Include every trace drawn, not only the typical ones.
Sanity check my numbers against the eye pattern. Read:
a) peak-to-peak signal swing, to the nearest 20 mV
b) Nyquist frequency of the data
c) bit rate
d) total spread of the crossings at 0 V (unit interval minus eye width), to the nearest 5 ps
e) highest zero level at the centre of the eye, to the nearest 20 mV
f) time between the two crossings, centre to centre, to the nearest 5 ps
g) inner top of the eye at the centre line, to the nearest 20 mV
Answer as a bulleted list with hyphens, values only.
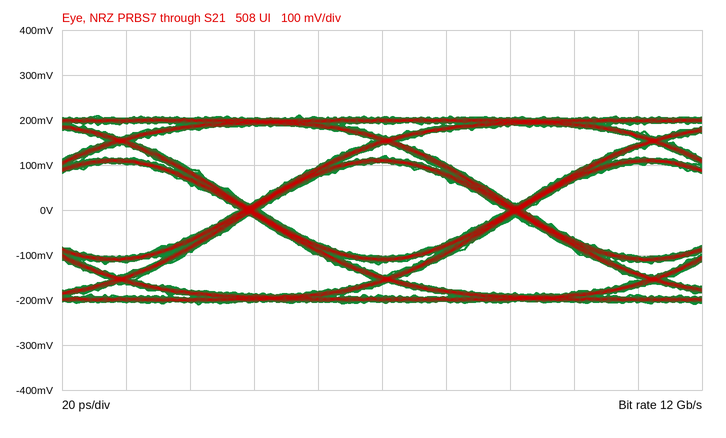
- 420 mV
- 6 GHz
- 12 Gb/s
- 5 ps
- -100 mV
- 85 ps
- 100 mV
